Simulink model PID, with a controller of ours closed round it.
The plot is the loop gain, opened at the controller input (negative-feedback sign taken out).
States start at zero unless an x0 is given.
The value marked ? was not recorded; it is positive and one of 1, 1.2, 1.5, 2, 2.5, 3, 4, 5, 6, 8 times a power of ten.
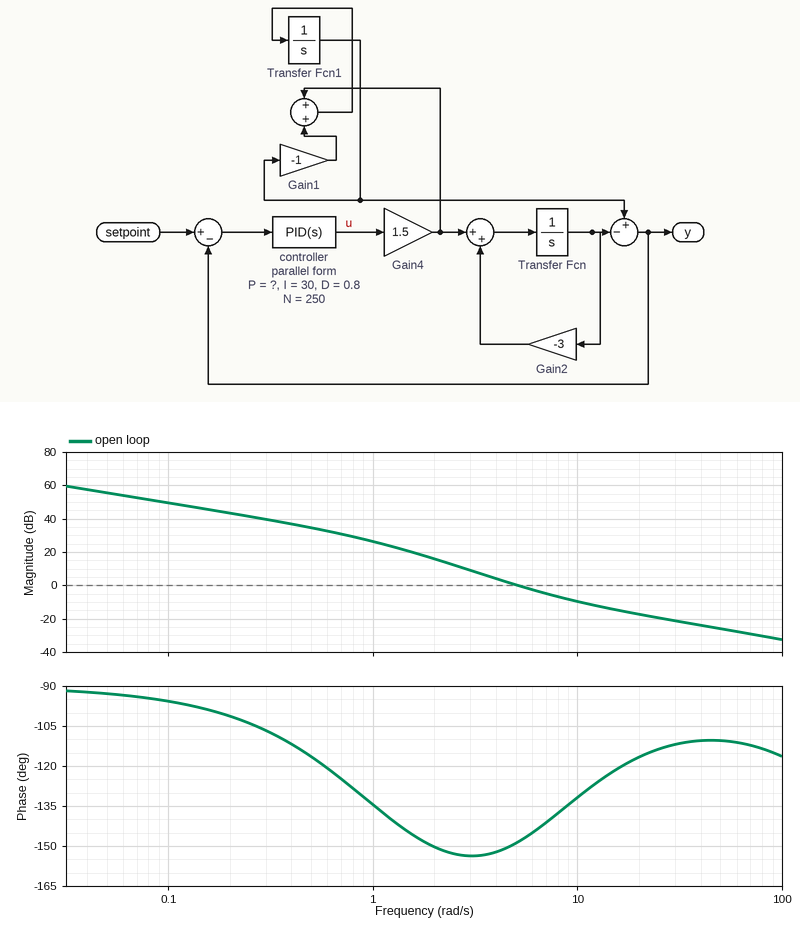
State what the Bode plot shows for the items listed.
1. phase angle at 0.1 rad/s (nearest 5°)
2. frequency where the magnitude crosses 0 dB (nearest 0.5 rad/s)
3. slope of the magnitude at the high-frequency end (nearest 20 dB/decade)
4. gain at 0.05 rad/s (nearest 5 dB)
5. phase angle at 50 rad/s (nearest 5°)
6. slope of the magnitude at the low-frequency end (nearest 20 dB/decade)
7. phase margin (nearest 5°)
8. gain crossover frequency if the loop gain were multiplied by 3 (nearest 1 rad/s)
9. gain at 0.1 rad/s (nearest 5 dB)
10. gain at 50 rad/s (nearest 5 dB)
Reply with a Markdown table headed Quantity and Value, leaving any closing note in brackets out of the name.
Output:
| Quantity | Value |
|---|---|
| phase angle at 0.1 rad/s | -95° |
| frequency where the magnitude crosses 0 dB | 5.0 rad/s |
| slope of the magnitude at the high-frequency end | -20 dB/decade |
| gain at 0.05 rad/s | 55 dB |
| phase angle at 50 rad/s | -110° |
| slope of the magnitude at the low-frequency end | -20 dB/decade |
| phase margin | 30° |
| gain crossover frequency if the loop gain were multiplied by 3 | 10 rad/s |
| gain at 0.1 rad/s | 50 dB |
| gain at 50 rad/s | -25 dB |
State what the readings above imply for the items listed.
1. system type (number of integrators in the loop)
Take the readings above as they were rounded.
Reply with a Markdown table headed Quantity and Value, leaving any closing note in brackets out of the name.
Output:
| Quantity | Value |
|---|---|
| system type | 1 |
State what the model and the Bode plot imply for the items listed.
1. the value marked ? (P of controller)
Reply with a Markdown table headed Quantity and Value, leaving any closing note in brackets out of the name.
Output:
| Quantity | Value |
|---|---|
| the value marked ? | 10 |
